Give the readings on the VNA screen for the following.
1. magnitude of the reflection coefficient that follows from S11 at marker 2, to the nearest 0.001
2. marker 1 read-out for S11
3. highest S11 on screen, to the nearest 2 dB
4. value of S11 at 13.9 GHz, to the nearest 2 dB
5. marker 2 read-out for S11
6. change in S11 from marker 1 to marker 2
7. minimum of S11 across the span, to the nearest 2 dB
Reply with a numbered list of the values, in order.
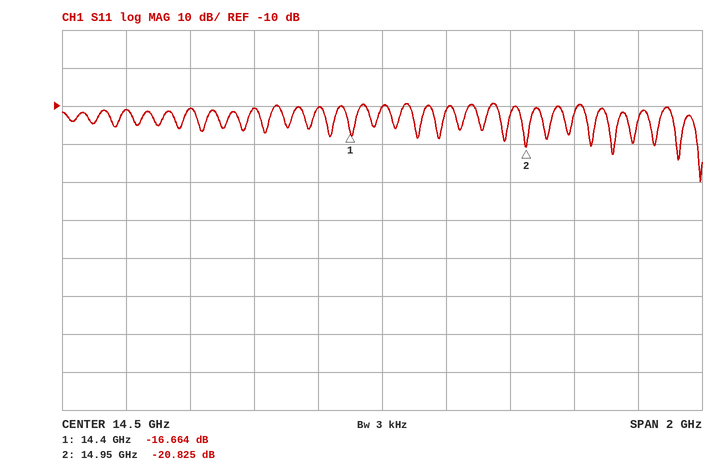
1. 0.091
2. -16.664 dB
3. -10 dB
4. -10 dB
5. -20.825 dB
6. -4.161 dB
7. -30 dB
